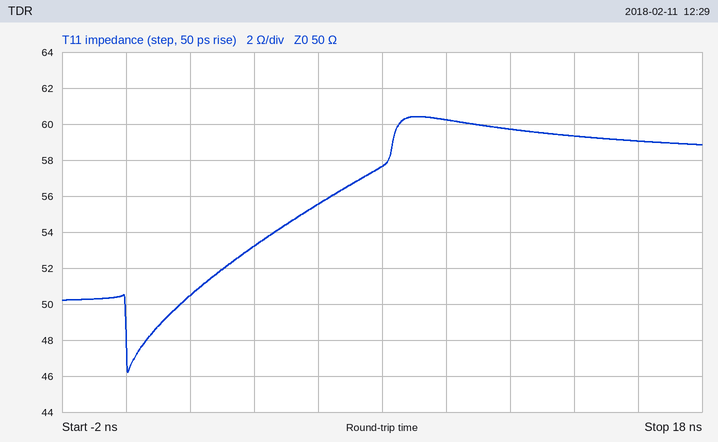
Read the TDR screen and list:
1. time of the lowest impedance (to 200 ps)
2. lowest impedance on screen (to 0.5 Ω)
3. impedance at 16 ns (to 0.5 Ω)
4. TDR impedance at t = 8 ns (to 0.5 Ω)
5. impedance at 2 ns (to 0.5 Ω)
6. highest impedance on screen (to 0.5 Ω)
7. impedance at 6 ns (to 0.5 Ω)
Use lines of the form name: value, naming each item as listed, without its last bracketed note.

time of the lowest impedance: 0.0 ns
lowest impedance on screen: 46.0 Ω
impedance at 16 ns: 59.0 Ω
TDR impedance at t = 8 ns: 57.5 Ω
impedance at 2 ns: 50.5 Ω
highest impedance on screen: 60.5 Ω
impedance at 6 ns: 55.5 Ω
